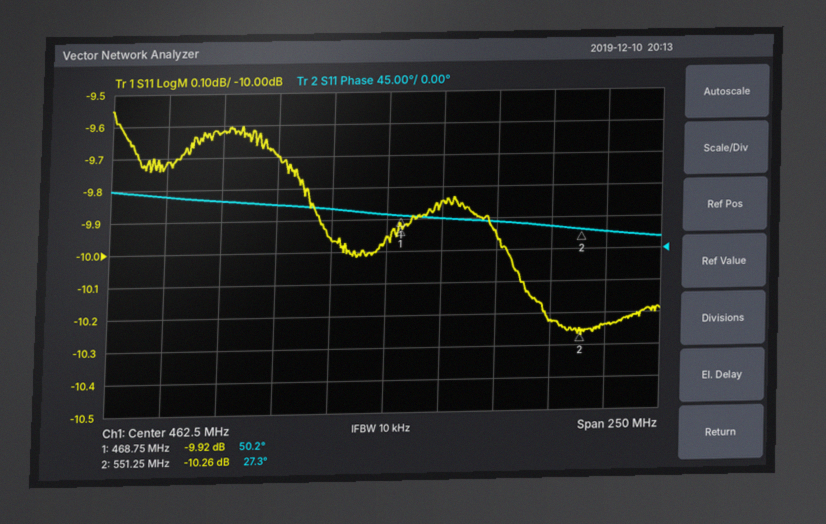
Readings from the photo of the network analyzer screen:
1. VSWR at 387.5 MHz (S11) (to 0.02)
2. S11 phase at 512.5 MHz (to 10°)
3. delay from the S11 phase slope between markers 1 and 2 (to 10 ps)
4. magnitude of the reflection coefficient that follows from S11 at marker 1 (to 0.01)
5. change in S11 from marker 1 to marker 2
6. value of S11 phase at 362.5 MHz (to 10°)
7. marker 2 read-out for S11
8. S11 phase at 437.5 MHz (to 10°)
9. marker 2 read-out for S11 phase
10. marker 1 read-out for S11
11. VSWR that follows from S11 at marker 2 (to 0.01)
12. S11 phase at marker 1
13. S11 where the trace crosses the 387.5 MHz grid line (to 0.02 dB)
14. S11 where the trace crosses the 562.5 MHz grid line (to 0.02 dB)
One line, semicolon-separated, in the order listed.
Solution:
1.98; 40°; 770 ps; 0.32; -0.34 dB; 80°; -10.26 dB; 60°; 27.3°; -9.92 dB; 1.89; 50.2°; -9.62 dB; -10.24 dB
